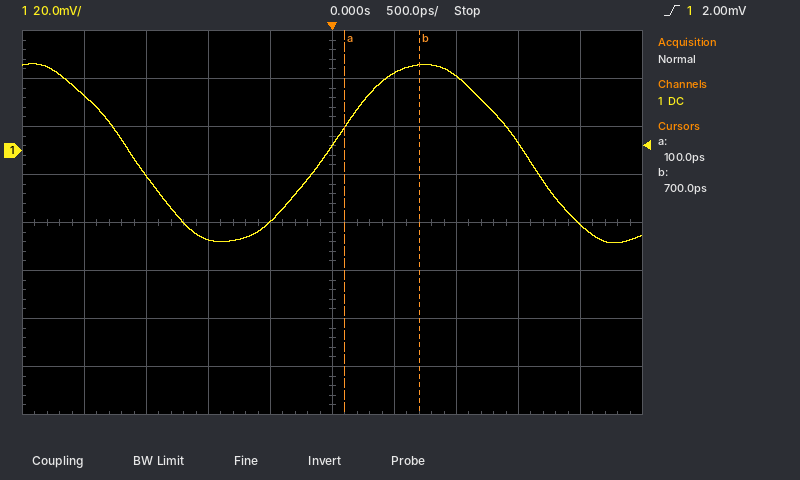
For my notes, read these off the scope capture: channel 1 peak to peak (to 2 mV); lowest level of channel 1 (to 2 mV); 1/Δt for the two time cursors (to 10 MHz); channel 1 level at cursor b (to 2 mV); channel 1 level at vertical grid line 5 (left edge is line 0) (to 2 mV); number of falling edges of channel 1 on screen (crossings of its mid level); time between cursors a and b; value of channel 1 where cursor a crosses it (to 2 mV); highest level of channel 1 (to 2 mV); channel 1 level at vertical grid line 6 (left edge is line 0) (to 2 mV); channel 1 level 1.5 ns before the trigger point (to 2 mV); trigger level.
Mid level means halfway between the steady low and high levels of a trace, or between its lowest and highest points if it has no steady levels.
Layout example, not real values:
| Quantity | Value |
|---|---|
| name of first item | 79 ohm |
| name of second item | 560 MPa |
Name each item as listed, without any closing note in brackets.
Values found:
| Quantity | Value |
|---|---|
| channel 1 peak to peak | 74 mV |
| lowest level of channel 1 | -38 mV |
| 1/Δt for the two time cursors | 1.67 GHz |
| channel 1 level at cursor b | 36 mV |
| channel 1 level at vertical grid line 5 (left edge is line 0) | 2 mV |
| number of falling edges of channel 1 on screen | 2 |
| time between cursors a and b | 600 ps |
| value of channel 1 where cursor a crosses it | 10 mV |
| highest level of channel 1 | 36 mV |
| channel 1 level at vertical grid line 6 (left edge is line 0) | 32 mV |
| channel 1 level 1.5 ns before the trigger point | -10 mV |
| trigger level | 2.00 mV |
